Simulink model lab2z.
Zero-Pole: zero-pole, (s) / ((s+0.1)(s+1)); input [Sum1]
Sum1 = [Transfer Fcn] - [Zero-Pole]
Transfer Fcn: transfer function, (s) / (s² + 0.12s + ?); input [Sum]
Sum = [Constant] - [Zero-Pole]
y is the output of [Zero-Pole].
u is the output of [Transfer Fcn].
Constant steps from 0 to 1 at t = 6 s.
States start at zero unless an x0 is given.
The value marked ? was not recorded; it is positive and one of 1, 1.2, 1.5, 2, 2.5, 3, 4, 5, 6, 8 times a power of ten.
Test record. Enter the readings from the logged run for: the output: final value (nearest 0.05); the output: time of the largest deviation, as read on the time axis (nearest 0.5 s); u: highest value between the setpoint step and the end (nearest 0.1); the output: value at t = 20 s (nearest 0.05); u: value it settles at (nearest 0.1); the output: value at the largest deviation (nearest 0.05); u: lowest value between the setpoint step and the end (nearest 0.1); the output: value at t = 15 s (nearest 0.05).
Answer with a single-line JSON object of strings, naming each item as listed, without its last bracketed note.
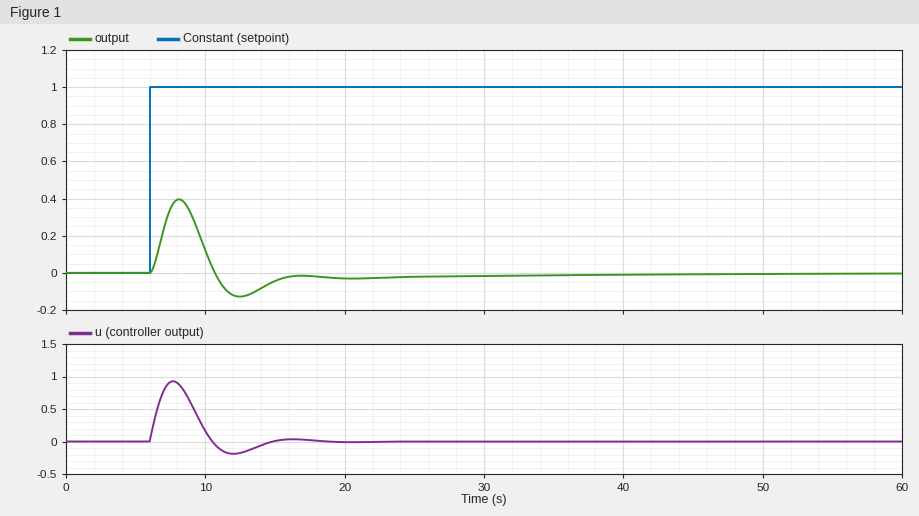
{"the output: final value": "0.00", "the output: time of the largest deviation, as read on the time axis": "8.0 s", "u: highest value between the setpoint step and the end": "0.9", "the output: value at t = 20 s": "-0.05", "u: value it settles at": "0.0", "the output: value at the largest deviation": "0.40", "u: lowest value between the setpoint step and the end": "-0.2", "the output: value at t = 15 s": "-0.05"}
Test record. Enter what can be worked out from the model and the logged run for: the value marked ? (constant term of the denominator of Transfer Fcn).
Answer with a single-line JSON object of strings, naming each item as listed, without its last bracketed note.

{"the value marked ?": "0.5"}
